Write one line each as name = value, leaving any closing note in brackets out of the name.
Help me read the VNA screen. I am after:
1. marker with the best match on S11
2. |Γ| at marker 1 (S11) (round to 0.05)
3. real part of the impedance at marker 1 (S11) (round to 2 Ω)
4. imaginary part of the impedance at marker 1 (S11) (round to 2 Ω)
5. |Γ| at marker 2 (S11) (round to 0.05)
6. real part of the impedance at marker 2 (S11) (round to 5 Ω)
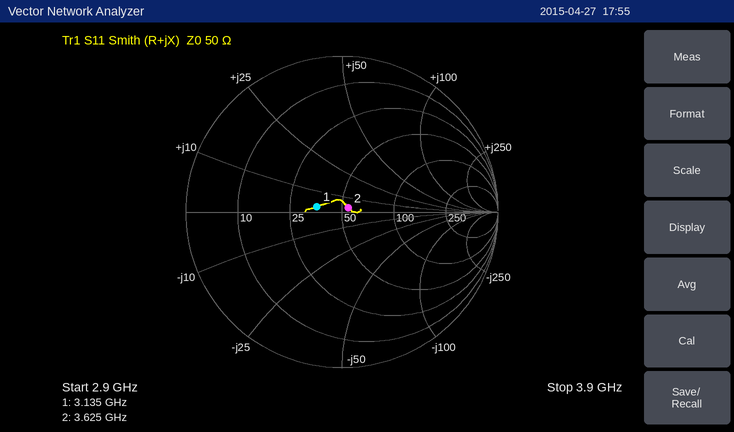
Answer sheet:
marker with the best match on S11 = marker 2
|Γ| at marker 1 (S11) = 0.15
real part of the impedance at marker 1 (S11) = 36 Ω
imaginary part of the impedance at marker 1 (S11) = +2 Ω
|Γ| at marker 2 (S11) = 0.05
real part of the impedance at marker 2 (S11) = 55 Ω
